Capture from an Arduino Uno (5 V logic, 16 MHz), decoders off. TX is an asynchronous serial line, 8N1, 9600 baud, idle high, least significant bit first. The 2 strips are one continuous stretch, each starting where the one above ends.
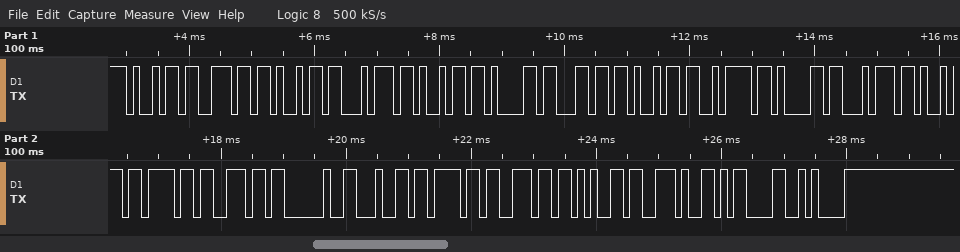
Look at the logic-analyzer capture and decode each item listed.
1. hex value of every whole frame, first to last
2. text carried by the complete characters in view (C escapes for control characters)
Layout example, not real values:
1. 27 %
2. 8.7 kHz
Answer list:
1. 0x69 0x6E 0x69 0x74 0x69 0x61 0x6C 0x69 0x7A 0x61 0x74 0x69 0x6F 0x6E 0x20 0x64 0x6F 0x6E 0x65 0x2E 0x0D 0x0A
2. "initialization done.\r\n"
